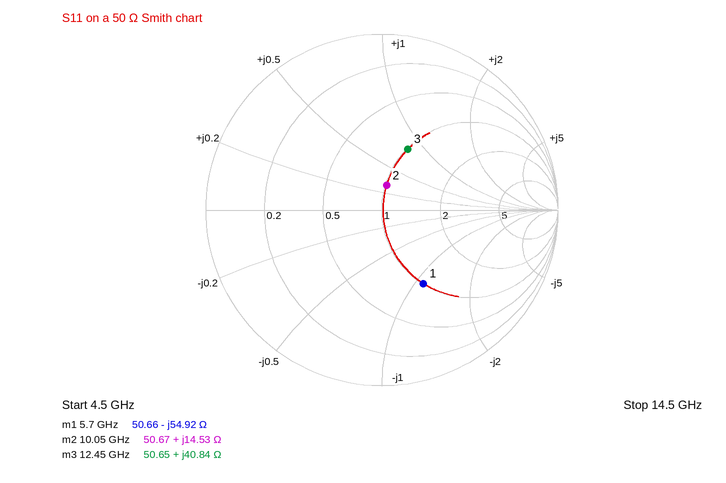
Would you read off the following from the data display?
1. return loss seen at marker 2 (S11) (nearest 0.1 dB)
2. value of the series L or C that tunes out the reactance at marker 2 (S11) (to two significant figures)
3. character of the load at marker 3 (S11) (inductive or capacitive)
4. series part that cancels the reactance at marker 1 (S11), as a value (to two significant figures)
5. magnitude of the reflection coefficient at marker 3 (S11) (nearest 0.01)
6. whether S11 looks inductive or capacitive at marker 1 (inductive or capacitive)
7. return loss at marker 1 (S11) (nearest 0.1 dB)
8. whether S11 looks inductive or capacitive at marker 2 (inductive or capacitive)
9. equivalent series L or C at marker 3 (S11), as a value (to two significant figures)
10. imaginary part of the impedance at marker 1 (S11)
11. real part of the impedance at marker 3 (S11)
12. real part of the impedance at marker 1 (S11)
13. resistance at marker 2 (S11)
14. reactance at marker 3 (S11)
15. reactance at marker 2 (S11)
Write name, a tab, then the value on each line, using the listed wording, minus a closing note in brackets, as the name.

return loss seen at marker 2 (S11)	16.9 dB
value of the series L or C that tunes out the reactance at marker 2 (S11)	1.1 pF
character of the load at marker 3 (S11)	inductive
series part that cancels the reactance at marker 1 (S11), as a value	1.5 nH
magnitude of the reflection coefficient at marker 3 (S11)	0.38
whether S11 looks inductive or capacitive at marker 1	capacitive
return loss at marker 1 (S11)	6.4 dB
whether S11 looks inductive or capacitive at marker 2	inductive
equivalent series L or C at marker 3 (S11), as a value	520 pH
imaginary part of the impedance at marker 1	-54.92 Ω
real part of the impedance at marker 3	50.65 Ω
real part of the impedance at marker 1	50.66 Ω
resistance at marker 2	50.67 Ω
reactance at marker 3	+40.84 Ω
reactance at marker 2	+14.53 Ω
